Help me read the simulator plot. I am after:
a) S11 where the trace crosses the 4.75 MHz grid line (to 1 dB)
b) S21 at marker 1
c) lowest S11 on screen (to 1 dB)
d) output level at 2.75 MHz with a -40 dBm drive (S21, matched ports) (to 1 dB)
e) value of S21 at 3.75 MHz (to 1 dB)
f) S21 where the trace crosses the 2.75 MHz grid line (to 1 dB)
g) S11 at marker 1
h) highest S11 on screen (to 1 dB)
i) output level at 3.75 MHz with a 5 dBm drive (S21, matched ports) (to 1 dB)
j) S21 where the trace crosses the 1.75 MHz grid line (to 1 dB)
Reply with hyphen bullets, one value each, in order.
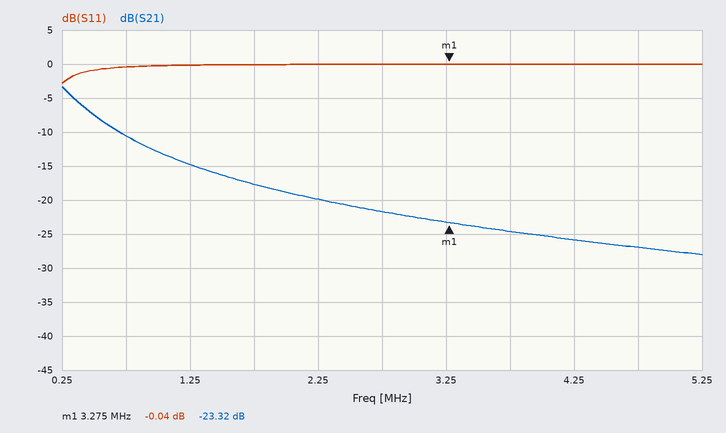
- 0 dB
- -23.32 dB
- -3 dB
- -62 dBm
- -25 dB
- -22 dB
- -0.04 dB
- 0 dB
- -20 dBm
- -18 dB
